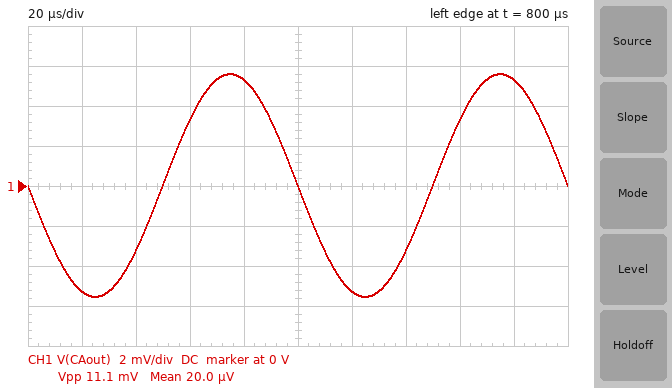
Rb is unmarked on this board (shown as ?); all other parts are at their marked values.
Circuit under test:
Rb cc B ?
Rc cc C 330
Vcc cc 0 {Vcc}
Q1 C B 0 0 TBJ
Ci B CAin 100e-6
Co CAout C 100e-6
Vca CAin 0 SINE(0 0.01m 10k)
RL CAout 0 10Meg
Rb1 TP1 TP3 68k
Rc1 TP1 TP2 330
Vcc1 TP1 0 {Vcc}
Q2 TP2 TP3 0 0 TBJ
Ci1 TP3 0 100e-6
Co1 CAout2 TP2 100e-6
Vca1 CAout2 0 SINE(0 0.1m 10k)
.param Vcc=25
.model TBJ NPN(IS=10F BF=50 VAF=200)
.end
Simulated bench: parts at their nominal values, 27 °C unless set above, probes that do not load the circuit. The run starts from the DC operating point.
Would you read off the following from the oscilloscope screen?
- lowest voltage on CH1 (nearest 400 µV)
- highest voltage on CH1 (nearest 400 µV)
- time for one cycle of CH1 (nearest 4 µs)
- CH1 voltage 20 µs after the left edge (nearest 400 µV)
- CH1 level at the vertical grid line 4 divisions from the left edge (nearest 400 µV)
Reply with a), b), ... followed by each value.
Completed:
a) -5.6 mV
b) 5.6 mV
c) 100 µs
d) -5.2 mV
e) 5.2 mV
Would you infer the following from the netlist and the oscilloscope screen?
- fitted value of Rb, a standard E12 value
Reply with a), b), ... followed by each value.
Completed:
a) 27 kΩ
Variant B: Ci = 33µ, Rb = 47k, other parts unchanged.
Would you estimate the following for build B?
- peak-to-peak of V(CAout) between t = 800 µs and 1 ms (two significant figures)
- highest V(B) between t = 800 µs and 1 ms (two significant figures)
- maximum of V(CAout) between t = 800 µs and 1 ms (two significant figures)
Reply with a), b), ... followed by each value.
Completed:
a) 6.8 mV
b) 740 mV
c) 3.4 mV
